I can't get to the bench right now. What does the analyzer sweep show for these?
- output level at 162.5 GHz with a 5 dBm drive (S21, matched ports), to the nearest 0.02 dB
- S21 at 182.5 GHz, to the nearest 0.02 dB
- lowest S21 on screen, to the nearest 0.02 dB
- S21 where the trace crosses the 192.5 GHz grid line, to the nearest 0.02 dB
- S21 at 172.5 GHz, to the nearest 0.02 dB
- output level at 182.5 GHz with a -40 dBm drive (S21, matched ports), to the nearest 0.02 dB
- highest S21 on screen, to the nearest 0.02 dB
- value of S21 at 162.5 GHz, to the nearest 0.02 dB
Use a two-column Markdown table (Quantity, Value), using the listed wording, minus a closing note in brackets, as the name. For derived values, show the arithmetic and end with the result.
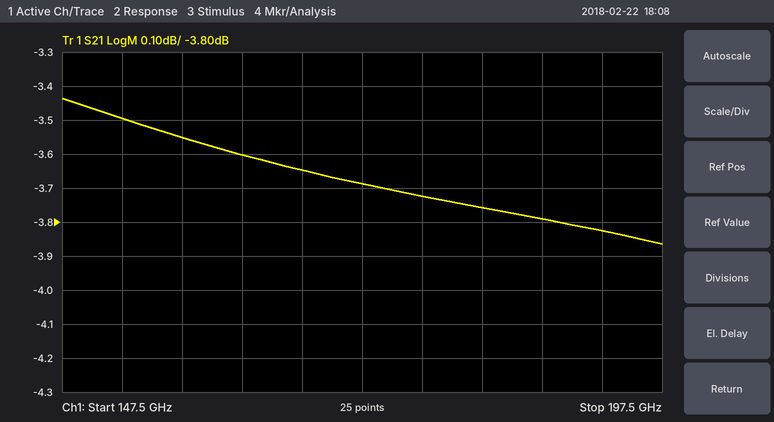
| Quantity | Value |
|---|---|
| output level at 162.5 GHz with a 5 dBm drive (S21, matched ports), to the nearest 0.02 dB | 5 dBm + (-3.60 dB) = 1.40 dBm |
| S21 at 182.5 GHz, to the nearest 0.02 dB | -3.76 dB |
| lowest S21 on screen, to the nearest 0.02 dB | -3.86 dB |
| S21 where the trace crosses the 192.5 GHz grid line, to the nearest 0.02 dB | -3.82 dB |
| S21 at 172.5 GHz, to the nearest 0.02 dB | -3.68 dB |
| output level at 182.5 GHz with a -40 dBm drive (S21, matched ports), to the nearest 0.02 dB | -40 dBm + (-3.76 dB) = -43.76 dBm |
| highest S21 on screen, to the nearest 0.02 dB | -3.44 dB |
| value of S21 at 162.5 GHz, to the nearest 0.02 dB | -3.60 dB |
